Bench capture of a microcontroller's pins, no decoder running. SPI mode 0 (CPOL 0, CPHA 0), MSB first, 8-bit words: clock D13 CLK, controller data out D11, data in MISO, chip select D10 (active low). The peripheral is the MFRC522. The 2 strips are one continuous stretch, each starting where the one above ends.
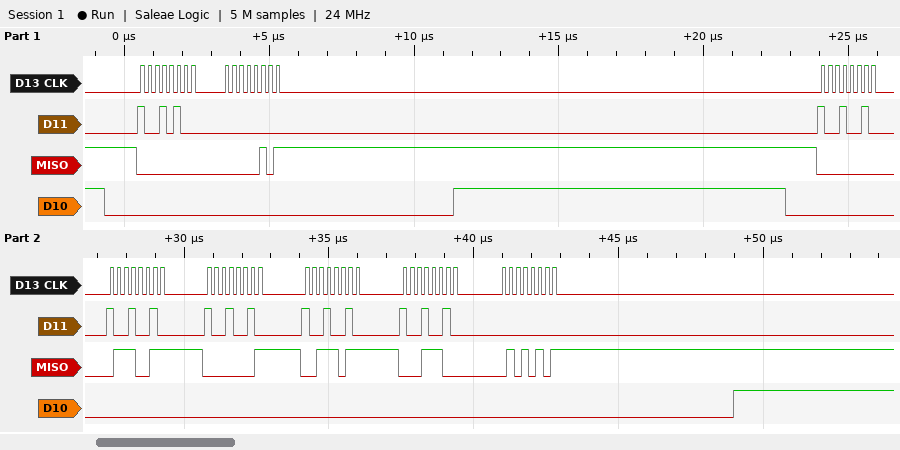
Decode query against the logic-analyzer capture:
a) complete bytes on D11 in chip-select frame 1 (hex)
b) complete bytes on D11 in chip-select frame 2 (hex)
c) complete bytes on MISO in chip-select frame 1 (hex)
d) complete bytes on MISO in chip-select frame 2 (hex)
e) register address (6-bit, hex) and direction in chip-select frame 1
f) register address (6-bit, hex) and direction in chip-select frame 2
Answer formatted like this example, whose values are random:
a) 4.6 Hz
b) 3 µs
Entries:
a) 94 00
b) 92 92 92 92 92 00
c) 00 05
d) 00 73 01 3B 1C 55
e) 0x0A read
f) 0x09 read
